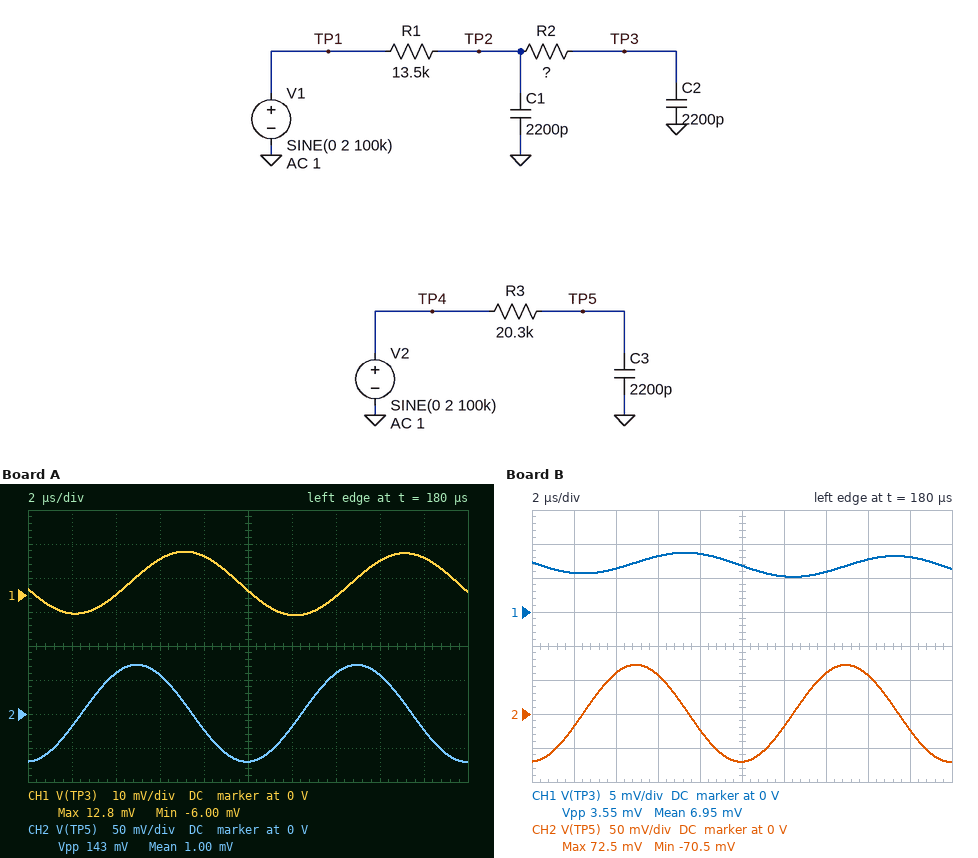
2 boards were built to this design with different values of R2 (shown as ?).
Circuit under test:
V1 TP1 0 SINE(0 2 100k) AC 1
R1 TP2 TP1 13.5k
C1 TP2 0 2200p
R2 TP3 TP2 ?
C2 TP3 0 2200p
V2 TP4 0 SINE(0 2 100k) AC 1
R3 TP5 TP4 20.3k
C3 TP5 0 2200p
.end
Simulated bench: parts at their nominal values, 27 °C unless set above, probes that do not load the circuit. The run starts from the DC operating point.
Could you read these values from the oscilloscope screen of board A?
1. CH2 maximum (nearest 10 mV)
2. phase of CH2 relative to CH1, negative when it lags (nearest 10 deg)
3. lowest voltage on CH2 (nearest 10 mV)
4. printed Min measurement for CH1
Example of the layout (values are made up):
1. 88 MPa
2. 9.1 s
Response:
1. 70 mV
2. 80 deg
3. -70 mV
4. -6.00 mV
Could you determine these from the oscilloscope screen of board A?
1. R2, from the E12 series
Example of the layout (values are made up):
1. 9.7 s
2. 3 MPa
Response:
1. 8.2 kΩ
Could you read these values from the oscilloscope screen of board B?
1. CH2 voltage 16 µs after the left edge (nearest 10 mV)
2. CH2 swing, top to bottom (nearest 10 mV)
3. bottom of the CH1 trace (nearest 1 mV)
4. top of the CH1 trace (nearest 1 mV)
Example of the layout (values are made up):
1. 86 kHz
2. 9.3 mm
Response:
1. 60 mV
2. 140 mV
3. 5 mV
4. 9 mV
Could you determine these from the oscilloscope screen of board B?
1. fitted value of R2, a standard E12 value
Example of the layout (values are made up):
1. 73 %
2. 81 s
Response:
1. 47 kΩ
